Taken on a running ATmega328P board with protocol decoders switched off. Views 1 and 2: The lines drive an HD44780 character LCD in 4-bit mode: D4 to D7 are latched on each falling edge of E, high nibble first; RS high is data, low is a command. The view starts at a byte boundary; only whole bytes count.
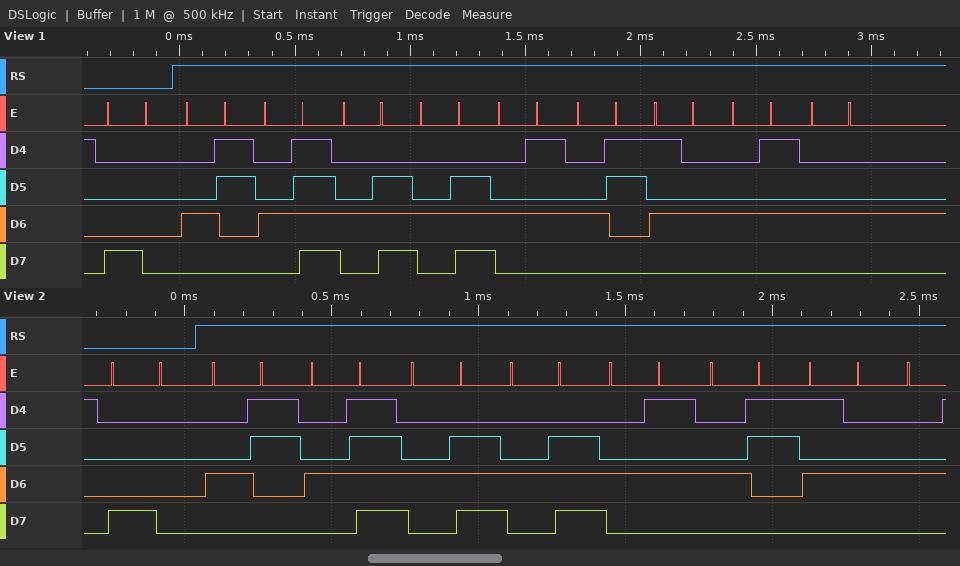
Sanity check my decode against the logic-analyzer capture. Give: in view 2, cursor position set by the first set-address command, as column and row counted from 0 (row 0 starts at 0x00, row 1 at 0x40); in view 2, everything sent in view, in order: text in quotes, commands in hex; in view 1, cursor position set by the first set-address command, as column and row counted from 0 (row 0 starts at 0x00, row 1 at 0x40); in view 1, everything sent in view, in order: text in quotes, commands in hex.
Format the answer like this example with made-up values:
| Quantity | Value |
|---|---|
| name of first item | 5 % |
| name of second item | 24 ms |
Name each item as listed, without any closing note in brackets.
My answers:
| Quantity | Value |
|---|---|
| in view 2, cursor position set by the first set-address command, as column and row counted from 0 | column 0, row 0 |
| in view 2, everything sent in view, in order: text in quotes, commands in hex | 0x80 "CONNECT" |
| in view 1, cursor position set by the first set-address command, as column and row counted from 0 | column 0, row 0 |
| in view 1, everything sent in view, in order: text in quotes, commands in hex | 0x80 "CONNECTED" |
